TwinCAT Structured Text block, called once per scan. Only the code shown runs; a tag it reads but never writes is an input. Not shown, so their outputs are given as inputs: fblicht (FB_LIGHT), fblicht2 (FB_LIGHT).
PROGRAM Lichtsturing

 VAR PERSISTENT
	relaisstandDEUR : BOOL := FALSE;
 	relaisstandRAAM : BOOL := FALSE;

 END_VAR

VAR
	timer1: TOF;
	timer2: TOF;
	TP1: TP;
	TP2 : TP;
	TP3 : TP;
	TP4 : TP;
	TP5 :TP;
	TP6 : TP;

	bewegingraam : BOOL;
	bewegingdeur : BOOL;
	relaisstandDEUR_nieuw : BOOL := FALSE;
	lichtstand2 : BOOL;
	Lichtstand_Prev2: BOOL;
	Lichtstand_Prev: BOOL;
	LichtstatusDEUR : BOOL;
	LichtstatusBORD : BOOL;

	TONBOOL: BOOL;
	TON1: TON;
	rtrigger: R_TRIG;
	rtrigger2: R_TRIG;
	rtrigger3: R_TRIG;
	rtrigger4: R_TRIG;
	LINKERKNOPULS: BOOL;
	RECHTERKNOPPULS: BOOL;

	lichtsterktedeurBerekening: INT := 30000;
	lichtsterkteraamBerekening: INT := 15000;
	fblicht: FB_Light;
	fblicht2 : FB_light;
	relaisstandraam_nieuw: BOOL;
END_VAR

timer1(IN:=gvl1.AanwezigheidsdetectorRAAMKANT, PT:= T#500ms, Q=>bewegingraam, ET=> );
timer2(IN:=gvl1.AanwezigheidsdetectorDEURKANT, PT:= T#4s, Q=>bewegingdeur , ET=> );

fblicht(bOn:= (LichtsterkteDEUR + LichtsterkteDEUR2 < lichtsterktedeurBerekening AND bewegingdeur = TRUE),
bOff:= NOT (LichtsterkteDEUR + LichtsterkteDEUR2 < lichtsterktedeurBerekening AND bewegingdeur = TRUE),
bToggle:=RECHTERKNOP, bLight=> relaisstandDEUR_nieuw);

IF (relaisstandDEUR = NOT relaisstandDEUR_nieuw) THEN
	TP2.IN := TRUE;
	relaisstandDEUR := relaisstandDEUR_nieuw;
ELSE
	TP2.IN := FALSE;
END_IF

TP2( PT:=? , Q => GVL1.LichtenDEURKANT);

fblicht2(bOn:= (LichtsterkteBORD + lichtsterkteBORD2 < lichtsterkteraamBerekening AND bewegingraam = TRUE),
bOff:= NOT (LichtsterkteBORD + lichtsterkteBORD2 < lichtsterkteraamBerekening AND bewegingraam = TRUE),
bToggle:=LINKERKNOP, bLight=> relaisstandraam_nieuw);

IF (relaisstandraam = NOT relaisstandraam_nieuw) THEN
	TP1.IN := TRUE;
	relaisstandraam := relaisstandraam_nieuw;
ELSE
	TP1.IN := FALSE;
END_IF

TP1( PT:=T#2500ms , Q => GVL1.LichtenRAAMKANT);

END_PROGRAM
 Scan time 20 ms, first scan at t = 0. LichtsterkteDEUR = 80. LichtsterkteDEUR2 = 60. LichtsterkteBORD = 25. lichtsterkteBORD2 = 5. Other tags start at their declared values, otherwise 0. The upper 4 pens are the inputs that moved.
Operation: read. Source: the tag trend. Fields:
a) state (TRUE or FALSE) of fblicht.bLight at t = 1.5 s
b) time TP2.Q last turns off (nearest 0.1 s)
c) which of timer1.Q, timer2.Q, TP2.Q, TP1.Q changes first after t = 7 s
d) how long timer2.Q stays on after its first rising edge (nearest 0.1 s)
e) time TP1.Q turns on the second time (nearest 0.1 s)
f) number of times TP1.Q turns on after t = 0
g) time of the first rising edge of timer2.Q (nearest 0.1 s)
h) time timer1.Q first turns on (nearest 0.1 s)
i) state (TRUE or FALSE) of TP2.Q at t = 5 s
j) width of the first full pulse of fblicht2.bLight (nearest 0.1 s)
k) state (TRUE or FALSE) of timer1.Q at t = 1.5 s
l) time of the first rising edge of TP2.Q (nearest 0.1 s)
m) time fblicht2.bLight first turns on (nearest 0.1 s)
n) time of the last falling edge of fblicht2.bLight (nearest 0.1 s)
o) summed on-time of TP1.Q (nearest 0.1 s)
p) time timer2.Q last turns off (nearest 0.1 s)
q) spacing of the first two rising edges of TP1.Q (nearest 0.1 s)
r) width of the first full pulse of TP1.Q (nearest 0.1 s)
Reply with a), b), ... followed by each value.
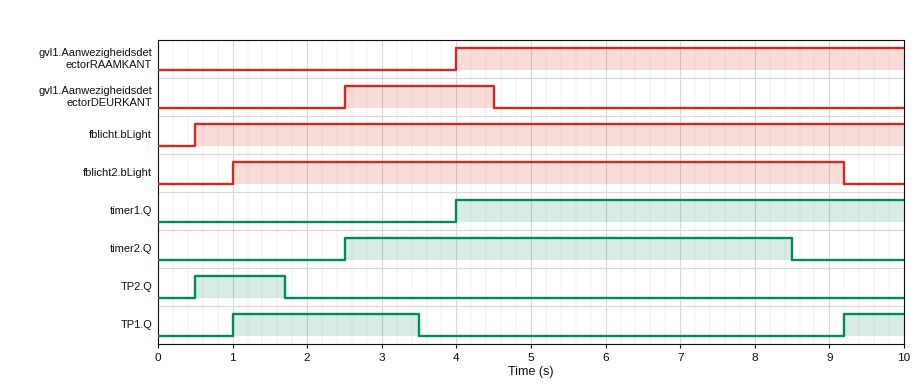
a) TRUE
b) 1.7 s
c) timer2.Q
d) 6.0 s
e) 9.2 s
f) 2
g) 2.5 s
h) 4.0 s
i) FALSE
j) 8.2 s
k) FALSE
l) 0.5 s
m) 1.0 s
n) 9.2 s
o) 3.3 s
p) 8.5 s
q) 8.2 s
r) 2.5 s
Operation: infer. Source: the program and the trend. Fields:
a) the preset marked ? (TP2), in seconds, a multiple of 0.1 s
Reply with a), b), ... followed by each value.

a) 1.2 s
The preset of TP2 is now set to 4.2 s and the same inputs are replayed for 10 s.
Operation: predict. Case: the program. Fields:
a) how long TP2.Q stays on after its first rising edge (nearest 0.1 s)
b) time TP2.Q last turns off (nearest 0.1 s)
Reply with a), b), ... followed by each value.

a) 4.2 s
b) 4.7 s
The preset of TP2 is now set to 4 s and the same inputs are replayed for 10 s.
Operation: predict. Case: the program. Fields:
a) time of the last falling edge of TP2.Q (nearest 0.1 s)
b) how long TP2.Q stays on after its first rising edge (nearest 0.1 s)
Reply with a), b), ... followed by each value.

a) 4.5 s
b) 4.0 s
